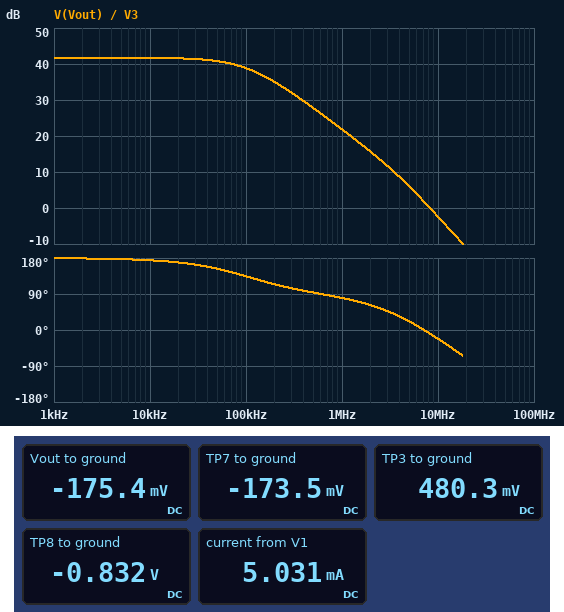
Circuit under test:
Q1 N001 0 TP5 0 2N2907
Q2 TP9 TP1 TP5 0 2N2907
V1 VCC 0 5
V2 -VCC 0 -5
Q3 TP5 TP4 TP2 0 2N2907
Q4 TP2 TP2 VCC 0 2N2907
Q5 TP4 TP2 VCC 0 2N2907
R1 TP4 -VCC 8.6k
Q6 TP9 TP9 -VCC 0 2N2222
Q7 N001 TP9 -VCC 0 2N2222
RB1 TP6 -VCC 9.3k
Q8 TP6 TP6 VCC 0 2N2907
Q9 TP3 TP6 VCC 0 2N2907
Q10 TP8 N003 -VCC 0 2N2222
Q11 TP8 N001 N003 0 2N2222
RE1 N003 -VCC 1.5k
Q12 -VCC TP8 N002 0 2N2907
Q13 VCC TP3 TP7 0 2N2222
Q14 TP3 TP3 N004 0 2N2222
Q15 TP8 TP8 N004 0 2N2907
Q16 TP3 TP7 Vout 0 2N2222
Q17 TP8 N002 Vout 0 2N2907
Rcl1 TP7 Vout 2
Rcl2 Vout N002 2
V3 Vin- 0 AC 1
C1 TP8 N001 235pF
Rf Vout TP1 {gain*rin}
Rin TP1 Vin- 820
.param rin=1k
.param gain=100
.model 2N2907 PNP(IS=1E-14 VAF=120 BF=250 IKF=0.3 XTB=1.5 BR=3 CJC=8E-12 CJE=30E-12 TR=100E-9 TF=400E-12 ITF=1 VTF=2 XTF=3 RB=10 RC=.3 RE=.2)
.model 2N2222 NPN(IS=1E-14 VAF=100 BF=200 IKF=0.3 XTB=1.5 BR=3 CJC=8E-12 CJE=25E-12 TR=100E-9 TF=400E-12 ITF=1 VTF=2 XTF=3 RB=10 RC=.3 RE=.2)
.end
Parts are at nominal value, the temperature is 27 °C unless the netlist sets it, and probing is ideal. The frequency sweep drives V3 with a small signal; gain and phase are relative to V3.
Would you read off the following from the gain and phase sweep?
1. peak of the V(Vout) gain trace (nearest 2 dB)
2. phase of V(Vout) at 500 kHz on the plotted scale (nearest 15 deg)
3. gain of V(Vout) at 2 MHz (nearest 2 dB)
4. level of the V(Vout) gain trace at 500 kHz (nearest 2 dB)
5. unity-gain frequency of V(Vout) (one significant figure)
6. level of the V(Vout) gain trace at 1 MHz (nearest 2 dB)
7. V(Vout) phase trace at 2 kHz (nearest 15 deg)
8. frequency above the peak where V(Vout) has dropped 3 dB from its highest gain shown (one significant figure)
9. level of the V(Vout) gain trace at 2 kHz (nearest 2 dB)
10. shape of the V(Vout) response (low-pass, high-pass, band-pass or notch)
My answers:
42 dB
90 deg
16 dB
28 dB
8 MHz
22 dB
180 deg
100 kHz
42 dB
low-pass
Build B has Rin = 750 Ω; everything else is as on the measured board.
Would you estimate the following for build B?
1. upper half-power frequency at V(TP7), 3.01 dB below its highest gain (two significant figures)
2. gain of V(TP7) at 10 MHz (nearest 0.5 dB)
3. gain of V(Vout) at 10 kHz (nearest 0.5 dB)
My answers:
94 kHz
-2.0 dB
42.5 dB
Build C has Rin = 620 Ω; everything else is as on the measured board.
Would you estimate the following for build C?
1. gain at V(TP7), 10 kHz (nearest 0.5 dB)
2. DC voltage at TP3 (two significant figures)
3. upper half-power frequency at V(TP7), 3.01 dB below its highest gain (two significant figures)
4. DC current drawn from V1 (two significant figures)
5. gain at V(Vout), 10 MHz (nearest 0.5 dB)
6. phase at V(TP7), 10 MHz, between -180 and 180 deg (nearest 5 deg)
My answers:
44.0 dB
490 mV
78 kHz
5.0 mA
-1.0 dB
-15 deg
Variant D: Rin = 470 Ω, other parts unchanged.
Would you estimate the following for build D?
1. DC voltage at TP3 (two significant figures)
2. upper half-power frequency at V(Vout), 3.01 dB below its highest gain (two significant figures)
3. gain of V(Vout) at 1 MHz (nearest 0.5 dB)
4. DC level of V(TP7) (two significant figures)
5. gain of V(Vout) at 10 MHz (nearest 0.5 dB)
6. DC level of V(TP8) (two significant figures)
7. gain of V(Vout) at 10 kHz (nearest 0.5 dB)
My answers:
490 mV
59 kHz
22.0 dB
-160 mV
0.5 dB
-820 mV
46.5 dB
